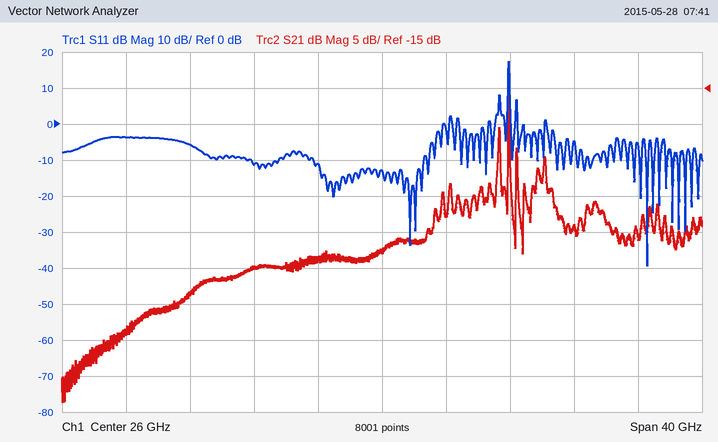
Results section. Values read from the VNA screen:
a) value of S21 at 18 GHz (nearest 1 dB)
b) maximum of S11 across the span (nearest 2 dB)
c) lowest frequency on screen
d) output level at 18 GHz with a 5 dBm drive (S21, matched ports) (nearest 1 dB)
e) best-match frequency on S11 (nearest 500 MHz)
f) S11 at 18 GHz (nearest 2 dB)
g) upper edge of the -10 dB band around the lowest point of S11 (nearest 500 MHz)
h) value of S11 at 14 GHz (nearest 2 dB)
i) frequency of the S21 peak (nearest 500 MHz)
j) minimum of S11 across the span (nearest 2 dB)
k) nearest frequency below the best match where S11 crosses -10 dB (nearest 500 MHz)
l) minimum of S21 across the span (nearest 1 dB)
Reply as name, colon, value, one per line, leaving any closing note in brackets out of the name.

value of S21 at 18 GHz: -40 dB
maximum of S11 across the span: 18 dB
lowest frequency on screen: 6 GHz
output level at 18 GHz with a 5 dBm drive (S21, matched ports): -35 dBm
best-match frequency on S11: 42.5 GHz
S11 at 18 GHz: -12 dB
upper edge of the -10 dB band around the lowest point of S11: 42.5 GHz
value of S11 at 14 GHz: -6 dB
frequency of the S21 peak: 34.0 GHz
minimum of S11 across the span: -40 dB
nearest frequency below the best match where S11 crosses -10 dB: 42.5 GHz
minimum of S21 across the span: -59 dB
